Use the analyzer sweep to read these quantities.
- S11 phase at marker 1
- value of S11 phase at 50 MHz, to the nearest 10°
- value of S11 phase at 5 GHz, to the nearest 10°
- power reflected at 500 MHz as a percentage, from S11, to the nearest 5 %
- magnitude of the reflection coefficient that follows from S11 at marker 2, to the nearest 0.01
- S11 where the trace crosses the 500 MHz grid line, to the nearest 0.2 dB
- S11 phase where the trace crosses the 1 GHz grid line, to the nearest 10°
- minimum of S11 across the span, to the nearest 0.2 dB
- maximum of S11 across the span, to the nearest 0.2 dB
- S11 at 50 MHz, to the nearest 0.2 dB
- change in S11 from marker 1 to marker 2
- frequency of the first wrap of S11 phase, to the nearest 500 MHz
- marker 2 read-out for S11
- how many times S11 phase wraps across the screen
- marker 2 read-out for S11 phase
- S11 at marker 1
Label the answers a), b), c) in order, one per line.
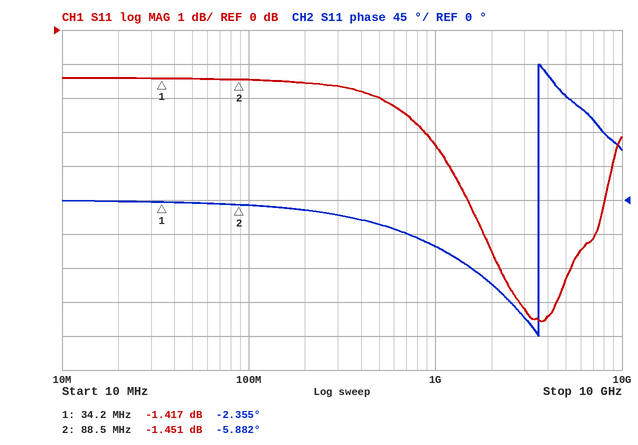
a) -2.355°
b) 0°
c) 140°
d) 65 %
e) 0.85
f) -2.0 dB
g) -60°
h) -8.6 dB
i) -1.4 dB
j) -1.4 dB
k) -0.034 dB
l) 3.5 GHz
m) -1.451 dB
n) 1
o) -5.882°
p) -1.417 dB
